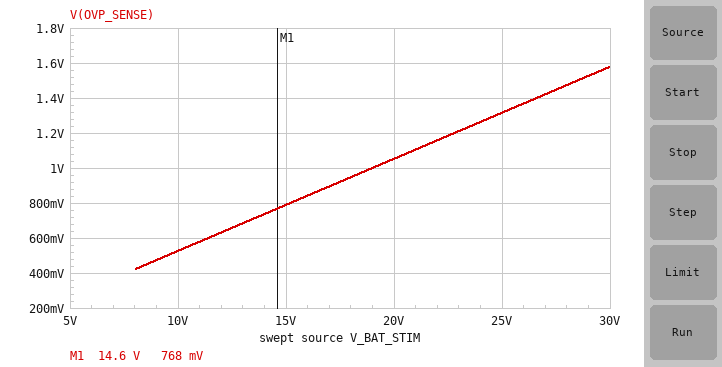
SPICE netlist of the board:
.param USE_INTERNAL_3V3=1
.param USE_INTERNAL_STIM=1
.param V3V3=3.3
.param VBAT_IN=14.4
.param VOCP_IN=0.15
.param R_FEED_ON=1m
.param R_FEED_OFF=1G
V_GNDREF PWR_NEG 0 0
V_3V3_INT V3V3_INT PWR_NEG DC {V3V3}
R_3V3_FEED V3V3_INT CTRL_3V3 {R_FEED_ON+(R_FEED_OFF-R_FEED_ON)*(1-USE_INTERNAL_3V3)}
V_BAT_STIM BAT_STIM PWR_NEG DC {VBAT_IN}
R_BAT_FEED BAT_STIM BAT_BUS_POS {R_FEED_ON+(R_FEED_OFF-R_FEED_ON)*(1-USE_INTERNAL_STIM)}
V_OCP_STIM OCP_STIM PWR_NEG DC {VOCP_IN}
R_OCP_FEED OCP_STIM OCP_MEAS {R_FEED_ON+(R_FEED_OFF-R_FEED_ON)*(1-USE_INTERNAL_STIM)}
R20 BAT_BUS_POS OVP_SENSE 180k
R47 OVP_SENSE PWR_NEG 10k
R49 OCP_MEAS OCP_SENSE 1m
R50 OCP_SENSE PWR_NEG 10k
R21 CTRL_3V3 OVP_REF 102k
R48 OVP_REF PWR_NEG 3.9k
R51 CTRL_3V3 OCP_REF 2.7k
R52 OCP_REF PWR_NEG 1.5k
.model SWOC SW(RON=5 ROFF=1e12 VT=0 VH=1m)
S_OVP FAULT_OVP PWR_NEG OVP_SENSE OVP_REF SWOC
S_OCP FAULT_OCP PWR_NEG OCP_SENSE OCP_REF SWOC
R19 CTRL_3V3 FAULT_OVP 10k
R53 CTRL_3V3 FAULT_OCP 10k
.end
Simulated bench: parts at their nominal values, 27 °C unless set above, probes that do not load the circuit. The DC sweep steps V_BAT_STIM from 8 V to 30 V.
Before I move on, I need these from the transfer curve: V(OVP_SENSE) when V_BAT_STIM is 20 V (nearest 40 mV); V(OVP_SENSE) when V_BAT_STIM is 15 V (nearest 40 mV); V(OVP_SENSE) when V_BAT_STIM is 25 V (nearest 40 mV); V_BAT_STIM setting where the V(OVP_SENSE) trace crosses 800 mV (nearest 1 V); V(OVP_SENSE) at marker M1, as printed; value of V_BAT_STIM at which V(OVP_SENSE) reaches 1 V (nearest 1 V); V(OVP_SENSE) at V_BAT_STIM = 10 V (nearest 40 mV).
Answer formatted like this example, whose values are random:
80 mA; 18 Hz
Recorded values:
1.04 V; 800 mV; 1.32 V; 15 V; 768 mV; 19 V; 520 mV
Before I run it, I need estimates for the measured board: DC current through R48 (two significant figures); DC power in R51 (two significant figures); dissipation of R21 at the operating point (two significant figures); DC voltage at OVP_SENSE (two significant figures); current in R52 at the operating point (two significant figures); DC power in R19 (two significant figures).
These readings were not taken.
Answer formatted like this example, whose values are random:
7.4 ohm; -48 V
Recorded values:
31 µA; 1.7 mW; 99 µW; 760 mV; 790 µA; 1.1 mW
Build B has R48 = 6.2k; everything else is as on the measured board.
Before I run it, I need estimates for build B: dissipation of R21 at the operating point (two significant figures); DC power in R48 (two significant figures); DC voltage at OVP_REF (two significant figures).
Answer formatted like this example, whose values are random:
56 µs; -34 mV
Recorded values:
95 µW; 5.8 µW; 190 mV
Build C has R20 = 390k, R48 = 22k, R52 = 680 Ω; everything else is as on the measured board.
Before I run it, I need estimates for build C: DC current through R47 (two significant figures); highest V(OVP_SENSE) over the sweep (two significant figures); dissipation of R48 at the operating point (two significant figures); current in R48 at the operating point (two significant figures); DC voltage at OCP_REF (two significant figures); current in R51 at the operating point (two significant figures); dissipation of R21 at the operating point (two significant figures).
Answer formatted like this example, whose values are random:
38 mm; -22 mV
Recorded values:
36 µA; 750 mV; 16 µW; 27 µA; 660 mV; 980 µA; 72 µW
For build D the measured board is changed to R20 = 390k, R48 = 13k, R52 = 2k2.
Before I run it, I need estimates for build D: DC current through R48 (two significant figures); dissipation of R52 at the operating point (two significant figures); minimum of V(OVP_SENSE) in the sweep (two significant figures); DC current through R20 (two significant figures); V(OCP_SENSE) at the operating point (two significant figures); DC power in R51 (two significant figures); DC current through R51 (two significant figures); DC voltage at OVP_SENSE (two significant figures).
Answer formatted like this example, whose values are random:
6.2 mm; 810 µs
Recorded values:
29 µA; 1.0 mW; 200 mV; 36 µA; 150 mV; 1.2 mW; 670 µA; 360 mV
